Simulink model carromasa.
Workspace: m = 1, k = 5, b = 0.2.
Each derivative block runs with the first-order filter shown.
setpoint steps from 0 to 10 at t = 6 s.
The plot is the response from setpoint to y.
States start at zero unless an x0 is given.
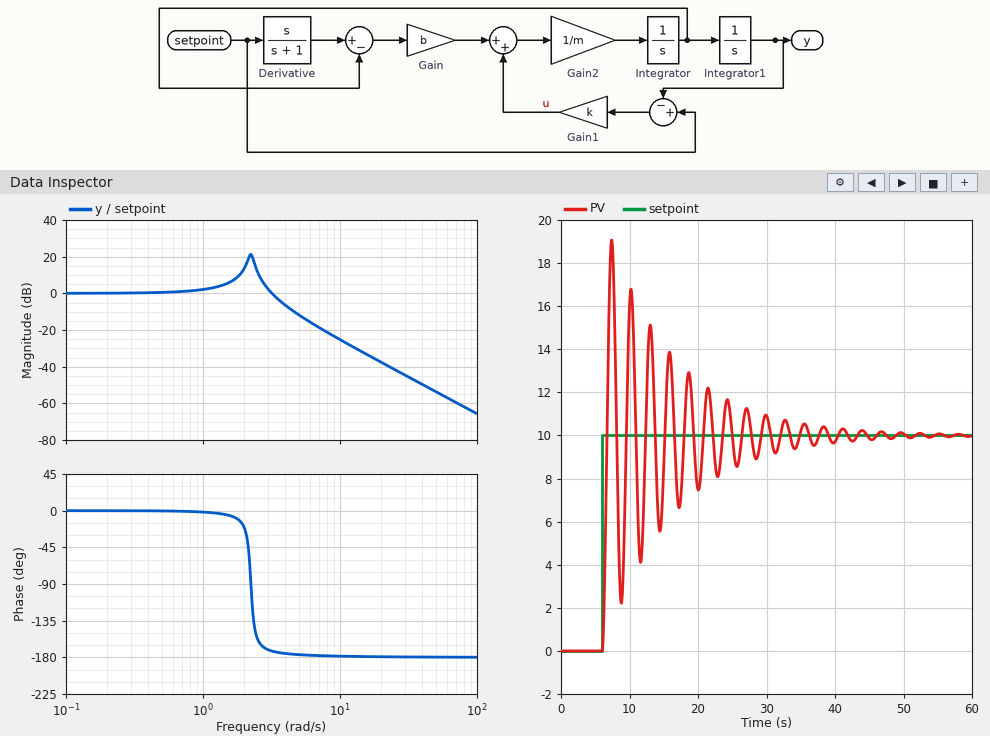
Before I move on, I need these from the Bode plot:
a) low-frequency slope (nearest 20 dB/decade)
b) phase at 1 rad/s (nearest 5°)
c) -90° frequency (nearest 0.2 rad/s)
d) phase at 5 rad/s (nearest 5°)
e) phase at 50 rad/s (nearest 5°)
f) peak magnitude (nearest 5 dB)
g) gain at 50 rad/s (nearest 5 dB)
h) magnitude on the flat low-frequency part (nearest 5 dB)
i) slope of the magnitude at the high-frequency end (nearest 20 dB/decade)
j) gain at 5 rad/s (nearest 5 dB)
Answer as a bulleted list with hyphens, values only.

- 0 dB/decade
- 0°
- 2.2 rad/s
- -175°
- -180°
- 20 dB
- -55 dB
- 0 dB
- -40 dB/decade
- -10 dB
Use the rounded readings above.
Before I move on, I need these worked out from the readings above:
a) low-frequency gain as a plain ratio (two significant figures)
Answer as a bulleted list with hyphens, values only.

- 1.0
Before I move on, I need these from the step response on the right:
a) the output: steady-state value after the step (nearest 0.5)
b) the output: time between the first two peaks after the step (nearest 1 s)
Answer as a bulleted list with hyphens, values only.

- 10.0
- 3 s
